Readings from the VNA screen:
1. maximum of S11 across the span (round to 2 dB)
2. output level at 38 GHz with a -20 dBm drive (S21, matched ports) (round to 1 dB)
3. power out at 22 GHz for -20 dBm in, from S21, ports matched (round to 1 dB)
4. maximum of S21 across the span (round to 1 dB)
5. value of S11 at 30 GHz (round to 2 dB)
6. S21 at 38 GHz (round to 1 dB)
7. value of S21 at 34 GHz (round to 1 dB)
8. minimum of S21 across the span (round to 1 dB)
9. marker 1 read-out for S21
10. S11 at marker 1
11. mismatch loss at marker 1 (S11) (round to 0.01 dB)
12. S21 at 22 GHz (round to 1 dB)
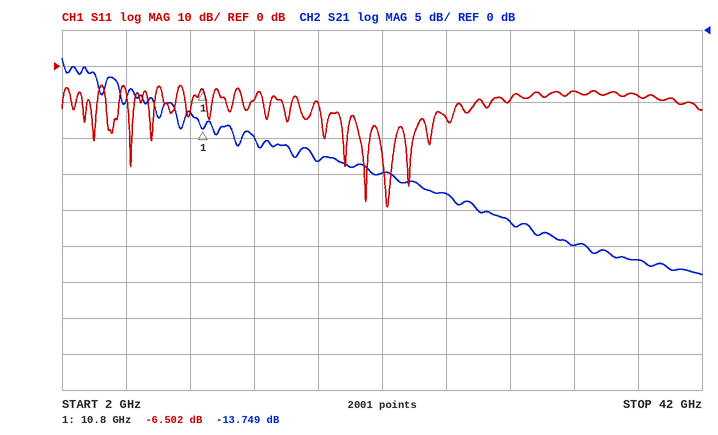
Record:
-6 dB
-52 dBm
-40 dBm
-4 dB
-10 dB
-32 dB
-30 dB
-34 dB
-13.749 dB
-6.502 dB
1.10 dB
-20 dB
